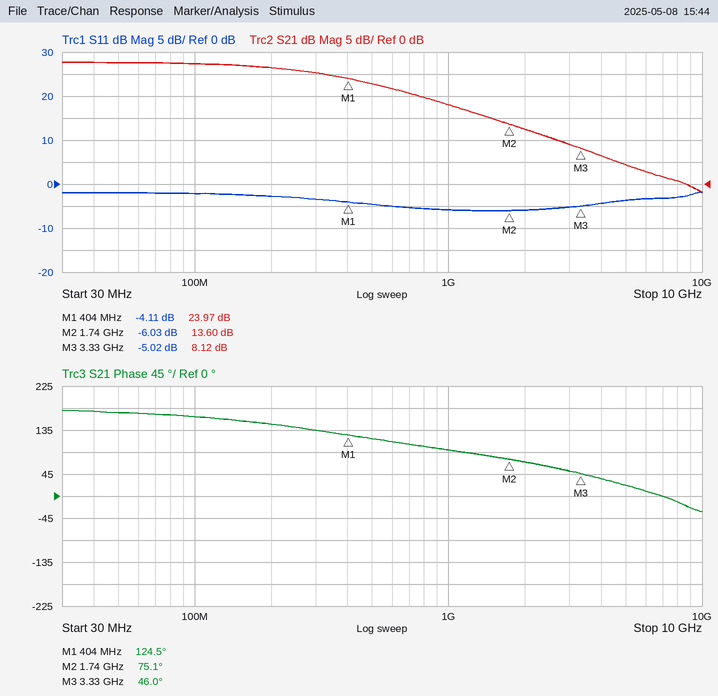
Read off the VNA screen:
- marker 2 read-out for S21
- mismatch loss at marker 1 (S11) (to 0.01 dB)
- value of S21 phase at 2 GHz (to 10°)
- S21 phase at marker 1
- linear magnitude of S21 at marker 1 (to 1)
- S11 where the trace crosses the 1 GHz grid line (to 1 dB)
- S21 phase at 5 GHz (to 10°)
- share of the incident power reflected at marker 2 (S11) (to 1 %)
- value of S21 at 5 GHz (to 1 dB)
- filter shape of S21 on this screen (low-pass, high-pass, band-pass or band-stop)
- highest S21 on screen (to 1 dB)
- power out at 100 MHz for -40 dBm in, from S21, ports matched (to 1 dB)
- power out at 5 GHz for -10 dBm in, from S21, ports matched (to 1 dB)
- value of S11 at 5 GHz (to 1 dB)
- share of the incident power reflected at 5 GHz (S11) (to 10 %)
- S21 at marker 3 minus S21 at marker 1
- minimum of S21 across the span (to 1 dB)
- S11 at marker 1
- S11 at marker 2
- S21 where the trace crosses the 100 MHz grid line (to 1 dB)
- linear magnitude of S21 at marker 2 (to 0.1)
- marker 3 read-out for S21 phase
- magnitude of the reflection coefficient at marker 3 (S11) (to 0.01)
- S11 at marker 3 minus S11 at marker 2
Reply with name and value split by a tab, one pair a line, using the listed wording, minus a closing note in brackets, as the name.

marker 2 read-out for S21	13.60 dB
mismatch loss at marker 1 (S11)	2.13 dB
value of S21 phase at 2 GHz	70°
S21 phase at marker 1	124.5°
linear magnitude of S21 at marker 1	16
S11 where the trace crosses the 1 GHz grid line	-6 dB
S21 phase at 5 GHz	20°
share of the incident power reflected at marker 2 (S11)	25 %
value of S21 at 5 GHz	4 dB
filter shape of S21 on this screen	low-pass
highest S21 on screen	28 dB
power out at 100 MHz for -40 dBm in, from S21, ports matched	-13 dBm
power out at 5 GHz for -10 dBm in, from S21, ports matched	-6 dBm
value of S11 at 5 GHz	-4 dB
share of the incident power reflected at 5 GHz (S11)	40 %
S21 at marker 3 minus S21 at marker 1	-15.85 dB
minimum of S21 across the span	-2 dB
S11 at marker 1	-4.11 dB
S11 at marker 2	-6.03 dB
S21 where the trace crosses the 100 MHz grid line	27 dB
linear magnitude of S21 at marker 2	4.8
marker 3 read-out for S21 phase	46.0°
magnitude of the reflection coefficient at marker 3 (S11)	0.56
S11 at marker 3 minus S11 at marker 2	1.01 dB
